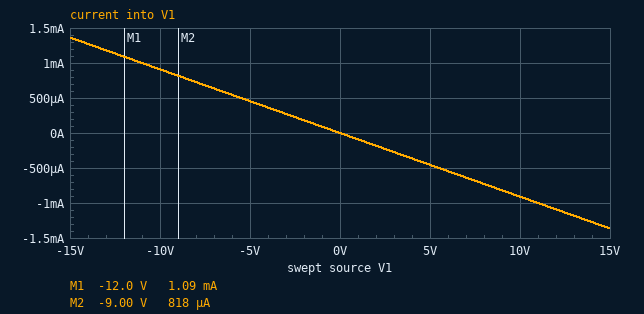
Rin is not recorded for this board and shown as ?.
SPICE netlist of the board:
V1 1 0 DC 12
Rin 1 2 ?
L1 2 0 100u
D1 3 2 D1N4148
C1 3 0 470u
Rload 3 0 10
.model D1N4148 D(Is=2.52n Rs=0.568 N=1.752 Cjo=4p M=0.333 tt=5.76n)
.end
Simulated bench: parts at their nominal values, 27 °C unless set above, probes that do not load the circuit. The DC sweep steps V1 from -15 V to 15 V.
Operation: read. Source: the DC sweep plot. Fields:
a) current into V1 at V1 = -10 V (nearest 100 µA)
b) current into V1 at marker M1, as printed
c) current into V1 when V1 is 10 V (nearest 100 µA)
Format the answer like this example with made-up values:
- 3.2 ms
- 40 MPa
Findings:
- 900 µA
- 1.09 mA
- -900 µA
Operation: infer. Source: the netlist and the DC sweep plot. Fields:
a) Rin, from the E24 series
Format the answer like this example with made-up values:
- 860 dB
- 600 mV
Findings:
- 11 kΩ
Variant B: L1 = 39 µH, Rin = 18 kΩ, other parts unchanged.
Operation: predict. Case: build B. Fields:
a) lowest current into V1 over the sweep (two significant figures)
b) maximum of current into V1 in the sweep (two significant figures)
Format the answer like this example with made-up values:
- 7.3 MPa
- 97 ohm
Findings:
- -830 µA
- 830 µA
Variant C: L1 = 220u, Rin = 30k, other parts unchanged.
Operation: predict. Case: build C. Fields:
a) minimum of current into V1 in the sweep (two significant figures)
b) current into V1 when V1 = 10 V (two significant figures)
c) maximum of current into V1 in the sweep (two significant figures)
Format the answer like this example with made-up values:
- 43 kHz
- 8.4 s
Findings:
- -500 µA
- -330 µA
- 500 µA
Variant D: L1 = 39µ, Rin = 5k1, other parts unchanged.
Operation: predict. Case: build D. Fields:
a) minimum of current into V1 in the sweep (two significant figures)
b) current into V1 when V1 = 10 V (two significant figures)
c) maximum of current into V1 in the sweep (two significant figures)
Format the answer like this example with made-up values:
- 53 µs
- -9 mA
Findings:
- -2.9 mA
- -2.0 mA
- 2.9 mA
